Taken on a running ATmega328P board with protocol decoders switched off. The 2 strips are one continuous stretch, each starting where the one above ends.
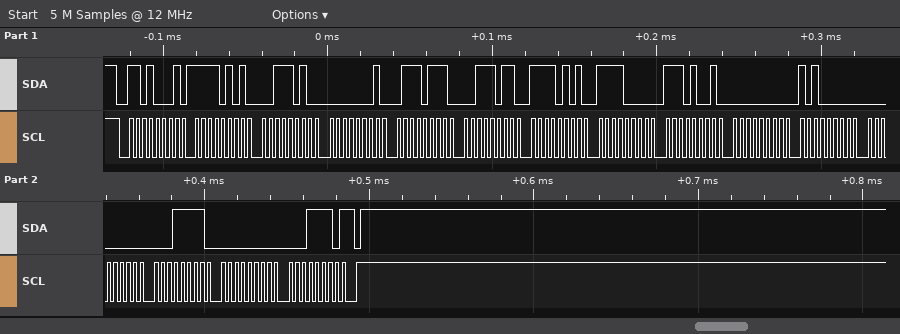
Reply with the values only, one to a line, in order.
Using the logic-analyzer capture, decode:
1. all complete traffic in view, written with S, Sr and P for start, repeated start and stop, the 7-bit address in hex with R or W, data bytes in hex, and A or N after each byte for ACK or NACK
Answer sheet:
S 68R A F5 A 3A A 01 A 77 A 3B A F5 A F0 A E9 A 00 A A0 A 00 A 1F A 00 A 1E N P
